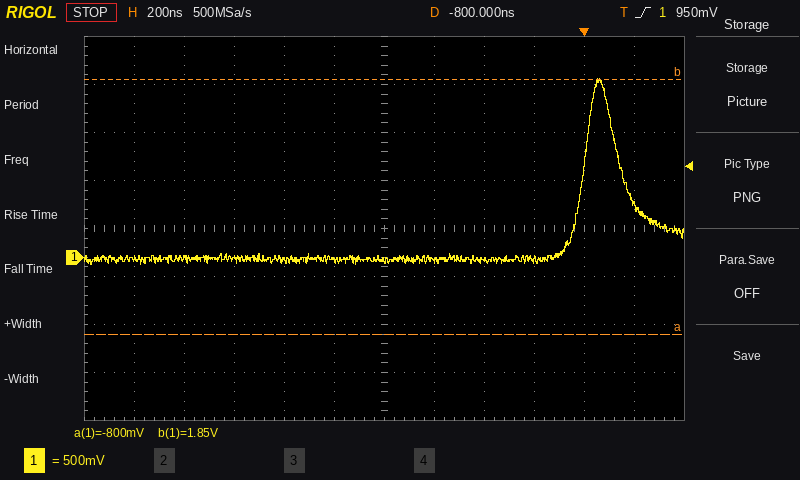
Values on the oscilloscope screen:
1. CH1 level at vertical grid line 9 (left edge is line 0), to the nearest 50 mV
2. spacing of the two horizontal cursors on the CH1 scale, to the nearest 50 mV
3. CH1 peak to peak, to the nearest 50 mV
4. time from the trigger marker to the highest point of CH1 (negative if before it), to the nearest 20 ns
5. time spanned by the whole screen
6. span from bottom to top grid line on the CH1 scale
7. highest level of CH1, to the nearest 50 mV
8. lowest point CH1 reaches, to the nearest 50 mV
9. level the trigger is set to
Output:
0 mV
2.65 V
1.95 V
+60 ns
2.4 µs
4 V
1.85 V
-100 mV
950 mV
